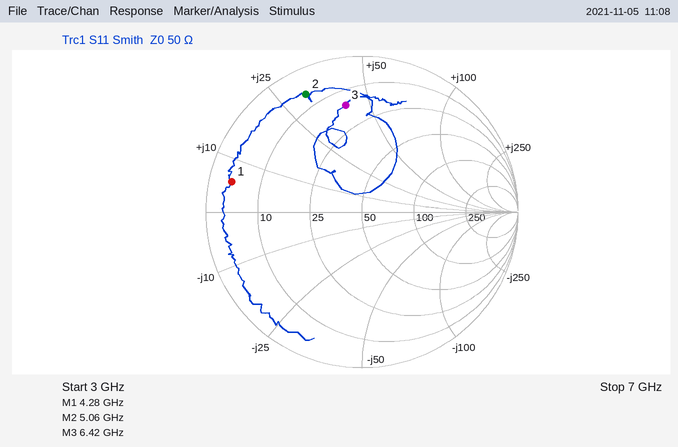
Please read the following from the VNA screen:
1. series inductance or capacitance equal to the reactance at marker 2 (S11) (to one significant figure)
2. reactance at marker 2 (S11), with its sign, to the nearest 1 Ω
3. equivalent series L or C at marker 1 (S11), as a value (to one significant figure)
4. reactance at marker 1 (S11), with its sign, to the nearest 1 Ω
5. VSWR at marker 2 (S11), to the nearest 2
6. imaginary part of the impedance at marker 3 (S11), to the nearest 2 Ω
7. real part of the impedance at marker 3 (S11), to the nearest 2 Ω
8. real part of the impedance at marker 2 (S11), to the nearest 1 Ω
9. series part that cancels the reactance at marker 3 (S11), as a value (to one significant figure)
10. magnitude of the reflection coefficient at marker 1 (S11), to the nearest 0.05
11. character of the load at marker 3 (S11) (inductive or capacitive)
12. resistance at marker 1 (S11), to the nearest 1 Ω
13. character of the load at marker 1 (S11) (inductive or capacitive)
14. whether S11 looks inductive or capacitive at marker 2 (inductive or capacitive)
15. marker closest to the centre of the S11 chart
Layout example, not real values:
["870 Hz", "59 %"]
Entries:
["1.0 nH", "+31 Ω", "200 pH", "+6 Ω", "12", "+40 Ω", "16 Ω", "6 Ω", "600 fF", "0.85", "inductive", "4 Ω", "inductive", "inductive", "marker 3"]
